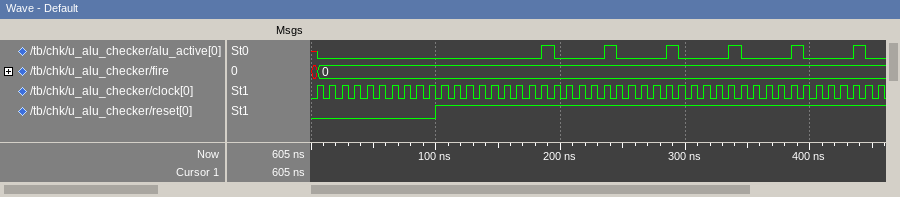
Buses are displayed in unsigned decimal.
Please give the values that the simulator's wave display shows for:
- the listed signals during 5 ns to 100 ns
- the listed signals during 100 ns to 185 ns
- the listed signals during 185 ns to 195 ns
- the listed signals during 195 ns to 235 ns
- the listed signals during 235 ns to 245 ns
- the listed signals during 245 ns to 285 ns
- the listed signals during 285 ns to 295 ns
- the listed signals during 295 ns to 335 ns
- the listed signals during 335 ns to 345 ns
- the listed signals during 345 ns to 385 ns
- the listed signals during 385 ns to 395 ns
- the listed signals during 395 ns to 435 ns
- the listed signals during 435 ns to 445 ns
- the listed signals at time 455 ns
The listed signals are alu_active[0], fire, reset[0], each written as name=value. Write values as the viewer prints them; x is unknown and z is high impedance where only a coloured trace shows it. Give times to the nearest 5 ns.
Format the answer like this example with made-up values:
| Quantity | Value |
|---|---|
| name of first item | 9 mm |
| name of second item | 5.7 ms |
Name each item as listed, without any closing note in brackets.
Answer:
| Quantity | Value |
|---|---|
| the listed signals during 5 ns to 100 ns | alu_active[0]=0, fire=0, reset[0]=0 |
| the listed signals during 100 ns to 185 ns | alu_active[0]=0, fire=0, reset[0]=1 |
| the listed signals during 185 ns to 195 ns | alu_active[0]=1, fire=0, reset[0]=1 |
| the listed signals during 195 ns to 235 ns | alu_active[0]=0, fire=0, reset[0]=1 |
| the listed signals during 235 ns to 245 ns | alu_active[0]=1, fire=0, reset[0]=1 |
| the listed signals during 245 ns to 285 ns | alu_active[0]=0, fire=0, reset[0]=1 |
| the listed signals during 285 ns to 295 ns | alu_active[0]=1, fire=0, reset[0]=1 |
| the listed signals during 295 ns to 335 ns | alu_active[0]=0, fire=0, reset[0]=1 |
| the listed signals during 335 ns to 345 ns | alu_active[0]=1, fire=0, reset[0]=1 |
| the listed signals during 345 ns to 385 ns | alu_active[0]=0, fire=0, reset[0]=1 |
| the listed signals during 385 ns to 395 ns | alu_active[0]=1, fire=0, reset[0]=1 |
| the listed signals during 395 ns to 435 ns | alu_active[0]=0, fire=0, reset[0]=1 |
| the listed signals during 435 ns to 445 ns | alu_active[0]=1, fire=0, reset[0]=1 |
| the listed signals at time 455 ns | alu_active[0]=0, fire=0, reset[0]=1 |
